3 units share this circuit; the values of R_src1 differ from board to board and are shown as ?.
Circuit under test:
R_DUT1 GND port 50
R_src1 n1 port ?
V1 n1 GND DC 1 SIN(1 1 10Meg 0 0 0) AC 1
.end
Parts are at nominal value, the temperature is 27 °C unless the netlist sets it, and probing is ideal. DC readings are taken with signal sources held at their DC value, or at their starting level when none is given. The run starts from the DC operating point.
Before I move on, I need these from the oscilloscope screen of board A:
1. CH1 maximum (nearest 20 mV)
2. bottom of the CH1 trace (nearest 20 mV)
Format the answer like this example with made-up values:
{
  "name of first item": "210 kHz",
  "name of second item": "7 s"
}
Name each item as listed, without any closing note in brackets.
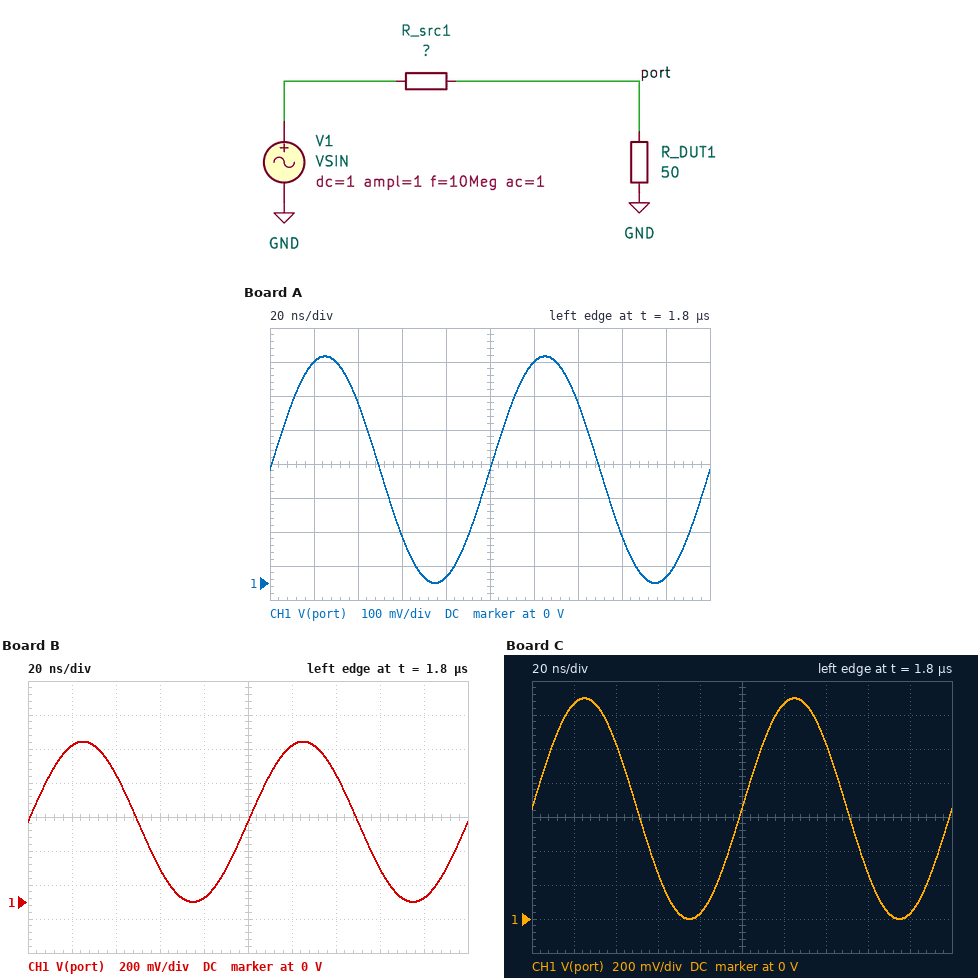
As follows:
{
  "CH1 maximum": "660 mV",
  "bottom of the CH1 trace": "0 V"
}
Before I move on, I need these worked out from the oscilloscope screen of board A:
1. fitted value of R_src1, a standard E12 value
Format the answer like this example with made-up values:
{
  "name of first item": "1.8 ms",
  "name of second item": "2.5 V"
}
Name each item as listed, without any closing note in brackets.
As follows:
{
  "fitted value of R_src1, a standard E12 value": "100 Ω"
}
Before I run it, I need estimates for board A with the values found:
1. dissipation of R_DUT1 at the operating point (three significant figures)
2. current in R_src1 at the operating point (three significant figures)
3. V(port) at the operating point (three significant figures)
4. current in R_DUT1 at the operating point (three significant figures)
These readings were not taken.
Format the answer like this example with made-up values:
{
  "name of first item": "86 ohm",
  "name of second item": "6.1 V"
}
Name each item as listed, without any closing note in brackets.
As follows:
{
  "dissipation of R_DUT1 at the operating point": "2.22 mW",
  "current in R_src1 at the operating point": "6.67 mA",
  "V(port) at the operating point": "333 mV",
  "current in R_DUT1 at the operating point": "6.67 mA"
}
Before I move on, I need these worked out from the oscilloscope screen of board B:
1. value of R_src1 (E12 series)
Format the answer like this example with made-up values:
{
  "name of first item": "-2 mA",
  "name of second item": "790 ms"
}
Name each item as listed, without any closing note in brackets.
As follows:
{
  "value of R_src1": "56 Ω"
}
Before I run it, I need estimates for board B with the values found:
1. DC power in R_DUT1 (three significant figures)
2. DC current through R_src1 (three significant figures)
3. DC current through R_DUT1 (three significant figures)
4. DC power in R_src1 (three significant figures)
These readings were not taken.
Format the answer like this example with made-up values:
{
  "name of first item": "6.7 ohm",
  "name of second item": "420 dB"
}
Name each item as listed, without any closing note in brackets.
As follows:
{
  "DC power in R_DUT1": "4.45 mW",
  "DC current through R_src1": "9.43 mA",
  "DC current through R_DUT1": "9.43 mA",
  "DC power in R_src1": "4.98 mW"
}
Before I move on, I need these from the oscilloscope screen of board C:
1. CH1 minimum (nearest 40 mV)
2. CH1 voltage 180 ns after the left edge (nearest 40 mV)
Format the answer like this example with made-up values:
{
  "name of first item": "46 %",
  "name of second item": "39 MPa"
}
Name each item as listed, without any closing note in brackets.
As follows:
{
  "CH1 minimum": "0 V",
  "CH1 voltage 180 ns after the left edge": "40 mV"
}
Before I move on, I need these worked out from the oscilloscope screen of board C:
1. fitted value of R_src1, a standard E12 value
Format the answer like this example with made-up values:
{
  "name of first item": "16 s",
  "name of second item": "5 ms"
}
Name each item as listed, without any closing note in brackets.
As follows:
{
  "fitted value of R_src1, a standard E12 value": "27 Ω"
}
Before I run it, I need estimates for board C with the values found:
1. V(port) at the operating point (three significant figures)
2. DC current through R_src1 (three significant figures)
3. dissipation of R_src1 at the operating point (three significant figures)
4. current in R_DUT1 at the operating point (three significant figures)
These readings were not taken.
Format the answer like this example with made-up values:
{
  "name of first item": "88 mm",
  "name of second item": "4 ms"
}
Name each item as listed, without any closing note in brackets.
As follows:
{
  "V(port) at the operating point": "649 mV",
  "DC current through R_src1": "13.0 mA",
  "dissipation of R_src1 at the operating point": "4.55 mW",
  "current in R_DUT1 at the operating point": "13.0 mA"
}
